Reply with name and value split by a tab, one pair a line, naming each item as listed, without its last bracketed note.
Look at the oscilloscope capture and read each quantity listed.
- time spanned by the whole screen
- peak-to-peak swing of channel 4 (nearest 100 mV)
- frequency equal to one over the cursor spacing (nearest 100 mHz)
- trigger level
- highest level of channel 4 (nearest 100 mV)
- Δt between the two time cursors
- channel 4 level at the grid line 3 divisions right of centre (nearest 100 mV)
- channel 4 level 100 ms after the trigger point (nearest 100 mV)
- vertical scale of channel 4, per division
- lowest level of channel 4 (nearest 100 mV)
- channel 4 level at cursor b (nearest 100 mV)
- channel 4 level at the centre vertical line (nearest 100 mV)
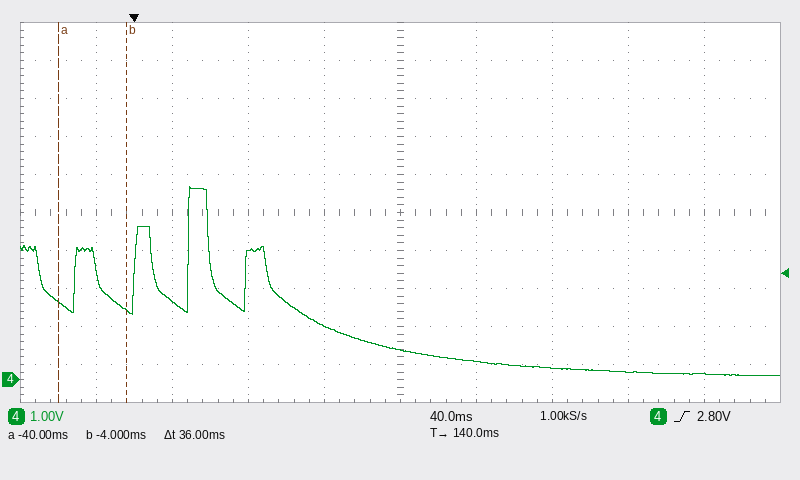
time spanned by the whole screen	400 ms
peak-to-peak swing of channel 4	5.0 V
frequency equal to one over the cursor spacing	27.8 Hz
trigger level	2.80 V
highest level of channel 4	5.1 V
Δt between the two time cursors	36 ms
channel 4 level at the grid line 3 divisions right of centre	200 mV
channel 4 level 100 ms after the trigger point	1.4 V
vertical scale of channel 4, per division	1 V
lowest level of channel 4	100 mV
channel 4 level at cursor b	1.8 V
channel 4 level at the centre vertical line	800 mV
